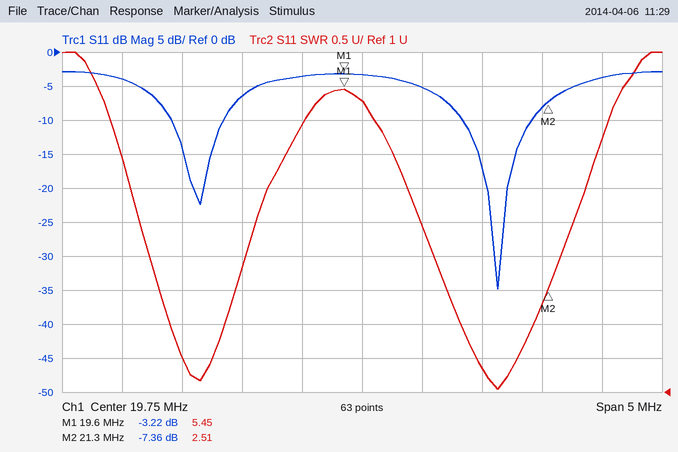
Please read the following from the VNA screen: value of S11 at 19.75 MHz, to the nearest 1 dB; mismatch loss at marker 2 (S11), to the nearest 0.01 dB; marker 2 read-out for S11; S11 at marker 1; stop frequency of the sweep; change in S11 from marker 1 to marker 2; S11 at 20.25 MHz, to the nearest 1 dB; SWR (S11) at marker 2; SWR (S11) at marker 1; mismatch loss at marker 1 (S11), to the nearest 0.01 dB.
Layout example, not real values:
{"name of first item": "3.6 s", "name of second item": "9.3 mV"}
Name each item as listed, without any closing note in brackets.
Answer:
{"value of S11 at 19.75 MHz, to the nearest 1 dB": "-3 dB", "mismatch loss at marker 2 (S11), to the nearest 0.01 dB": "0.88 dB", "marker 2 read-out for S11": "-7.36 dB", "S11 at marker 1": "-3.22 dB", "stop frequency of the sweep": "22.25 MHz", "change in S11 from marker 1 to marker 2": "-4.14 dB", "S11 at 20.25 MHz, to the nearest 1 dB": "-5 dB", "SWR (S11) at marker 2": "2.51", "SWR (S11) at marker 1": "5.45", "mismatch loss at marker 1 (S11), to the nearest 0.01 dB": "2.81 dB"}
